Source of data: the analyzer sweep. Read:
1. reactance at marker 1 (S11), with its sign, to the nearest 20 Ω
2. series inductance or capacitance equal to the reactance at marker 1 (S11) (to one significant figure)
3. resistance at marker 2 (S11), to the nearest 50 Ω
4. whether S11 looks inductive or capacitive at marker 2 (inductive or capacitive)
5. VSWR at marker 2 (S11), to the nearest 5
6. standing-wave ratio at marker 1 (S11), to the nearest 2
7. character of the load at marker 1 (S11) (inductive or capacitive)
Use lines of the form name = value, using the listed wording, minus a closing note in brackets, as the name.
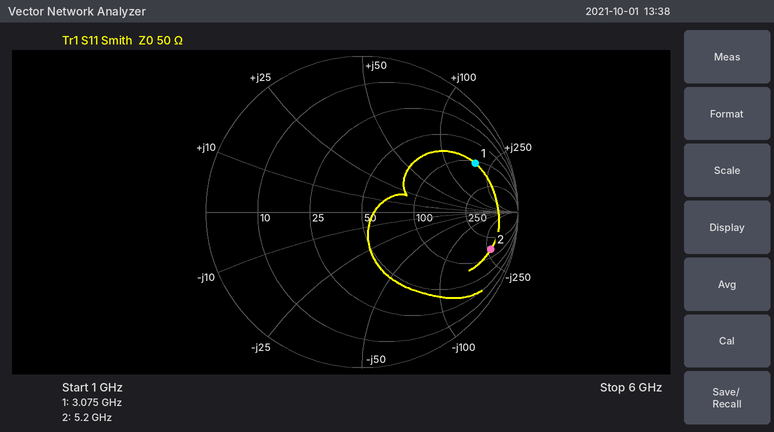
reactance at marker 1 (S11), with its sign, to the nearest 20 Ω = +180 Ω
series inductance or capacitance equal to the reactance at marker 1 (S11) = 9 nH
resistance at marker 2 (S11), to the nearest 50 Ω = 150 Ω
whether S11 looks inductive or capacitive at marker 2 = capacitive
VSWR at marker 2 (S11), to the nearest 5 = 15
standing-wave ratio at marker 1 (S11), to the nearest 2 = 8
character of the load at marker 1 (S11) = inductive
